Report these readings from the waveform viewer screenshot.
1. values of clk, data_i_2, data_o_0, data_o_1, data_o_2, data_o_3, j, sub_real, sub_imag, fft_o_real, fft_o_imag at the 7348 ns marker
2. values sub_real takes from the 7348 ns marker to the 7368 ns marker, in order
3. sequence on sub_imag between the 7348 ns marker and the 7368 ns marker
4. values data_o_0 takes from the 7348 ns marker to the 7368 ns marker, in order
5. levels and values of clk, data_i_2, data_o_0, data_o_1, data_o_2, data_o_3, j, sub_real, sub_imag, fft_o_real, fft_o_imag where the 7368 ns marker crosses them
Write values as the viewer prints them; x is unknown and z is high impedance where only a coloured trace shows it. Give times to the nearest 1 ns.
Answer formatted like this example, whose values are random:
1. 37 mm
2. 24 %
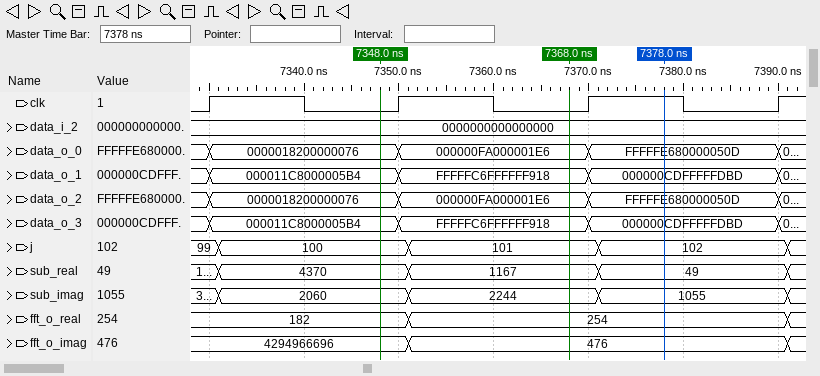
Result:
1. clk=0, data_i_2=0000000000000000, data_o_0=0000018200000076, data_o_1=000011C8000005B4, data_o_2=0000018200000076, data_o_3=000011C8000005B4, j=100, sub_real=4370, sub_imag=2060, fft_o_real=182, fft_o_imag=4294966696
2. 4370, 1167
3. 2060, 2244
4. 0000018200000076, 000000FA000001E6
5. clk=0, data_i_2=0000000000000000, data_o_0=000000FA000001E6, data_o_1=FFFFFC6FFFFFF918, data_o_2=000000FA000001E6, data_o_3=FFFFFC6FFFFFF918, j=101, sub_real=1167, sub_imag=2244, fft_o_real=254, fft_o_imag=476
